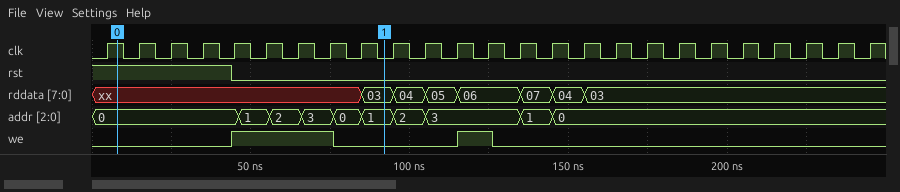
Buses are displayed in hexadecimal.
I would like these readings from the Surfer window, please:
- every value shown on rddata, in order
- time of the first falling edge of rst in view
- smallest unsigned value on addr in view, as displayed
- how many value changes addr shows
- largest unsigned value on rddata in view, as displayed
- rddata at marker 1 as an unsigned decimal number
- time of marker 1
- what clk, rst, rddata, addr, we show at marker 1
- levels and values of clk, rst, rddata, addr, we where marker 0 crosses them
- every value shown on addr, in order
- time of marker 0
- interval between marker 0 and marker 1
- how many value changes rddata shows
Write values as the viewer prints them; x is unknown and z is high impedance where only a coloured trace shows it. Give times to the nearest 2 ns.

xx, 03, 04, 05, 06, 07, 04, 03
44 ns
0
9
07
3
92 ns
clk=0, rst=0, rddata=03, addr=1, we=0
clk=1, rst=1, rddata=xx, addr=0, we=0
0, 1, 2, 3, 0, 1, 2, 3, 1, 0
8 ns
84 ns
7
